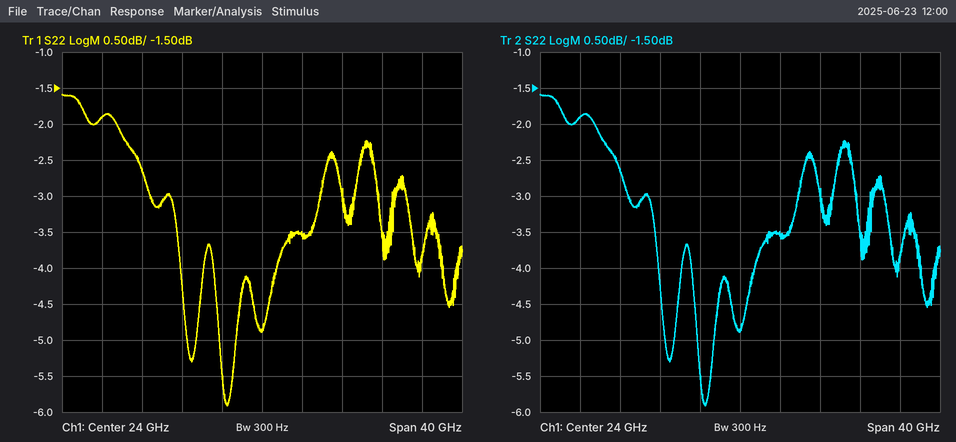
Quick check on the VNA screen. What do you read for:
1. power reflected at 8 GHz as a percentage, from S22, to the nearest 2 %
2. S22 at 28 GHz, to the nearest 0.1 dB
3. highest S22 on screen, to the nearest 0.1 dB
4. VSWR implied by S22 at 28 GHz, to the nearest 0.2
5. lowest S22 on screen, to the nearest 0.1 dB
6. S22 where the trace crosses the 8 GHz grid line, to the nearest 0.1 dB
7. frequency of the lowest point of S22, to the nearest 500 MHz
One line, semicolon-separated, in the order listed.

64 %; -3.5 dB; -1.6 dB; 5.0; -5.9 dB; -1.9 dB; 20.5 GHz
